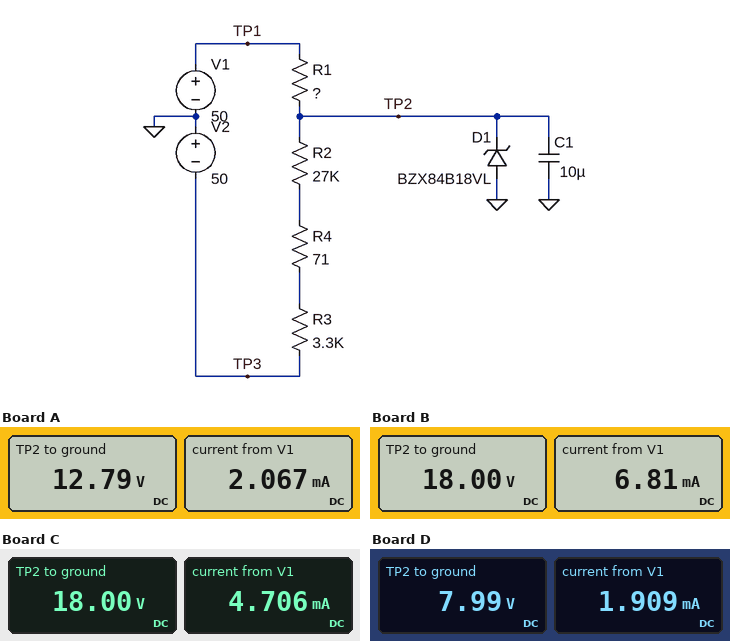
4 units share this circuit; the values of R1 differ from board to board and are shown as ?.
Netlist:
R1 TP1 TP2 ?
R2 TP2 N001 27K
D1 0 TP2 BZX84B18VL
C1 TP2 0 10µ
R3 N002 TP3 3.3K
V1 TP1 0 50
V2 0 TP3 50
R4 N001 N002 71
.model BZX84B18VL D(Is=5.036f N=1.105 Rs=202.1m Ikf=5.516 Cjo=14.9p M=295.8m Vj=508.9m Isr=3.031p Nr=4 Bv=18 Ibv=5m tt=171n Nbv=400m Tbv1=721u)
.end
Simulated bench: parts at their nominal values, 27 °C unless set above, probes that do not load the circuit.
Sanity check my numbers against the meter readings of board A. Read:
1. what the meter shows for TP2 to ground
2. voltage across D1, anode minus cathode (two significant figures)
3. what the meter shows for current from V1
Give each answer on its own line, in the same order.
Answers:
12.79 V
-13 V
2.067 mA
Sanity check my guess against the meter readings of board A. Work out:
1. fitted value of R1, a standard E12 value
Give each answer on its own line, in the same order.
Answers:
18 kΩ
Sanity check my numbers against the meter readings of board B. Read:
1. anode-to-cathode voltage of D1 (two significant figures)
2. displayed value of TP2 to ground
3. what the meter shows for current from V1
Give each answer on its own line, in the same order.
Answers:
-18 V
18.00 V
6.81 mA
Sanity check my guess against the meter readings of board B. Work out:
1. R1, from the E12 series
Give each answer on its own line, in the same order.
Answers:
4.7 kΩ
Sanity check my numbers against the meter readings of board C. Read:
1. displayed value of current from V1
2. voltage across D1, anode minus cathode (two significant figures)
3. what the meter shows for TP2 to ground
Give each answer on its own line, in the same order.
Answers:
4.706 mA
-18 V
18.00 V
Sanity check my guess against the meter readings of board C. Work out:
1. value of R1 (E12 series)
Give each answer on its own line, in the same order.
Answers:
6.8 kΩ
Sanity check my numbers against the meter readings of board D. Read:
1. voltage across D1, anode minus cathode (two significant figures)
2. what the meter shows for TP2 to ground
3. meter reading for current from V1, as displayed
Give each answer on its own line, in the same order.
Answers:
-8.0 V
7.99 V
1.909 mA
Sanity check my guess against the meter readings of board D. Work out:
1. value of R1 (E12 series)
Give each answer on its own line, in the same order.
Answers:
22 kΩ
